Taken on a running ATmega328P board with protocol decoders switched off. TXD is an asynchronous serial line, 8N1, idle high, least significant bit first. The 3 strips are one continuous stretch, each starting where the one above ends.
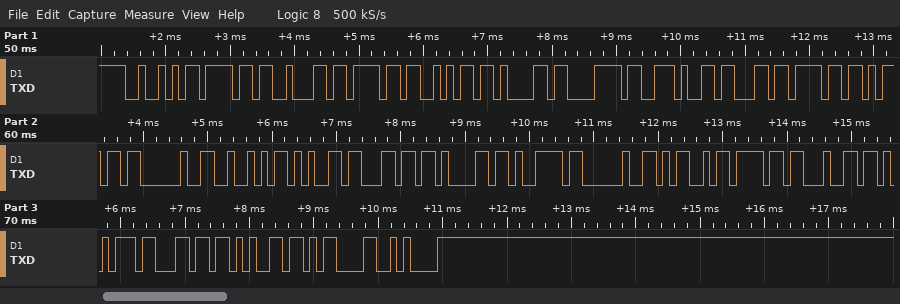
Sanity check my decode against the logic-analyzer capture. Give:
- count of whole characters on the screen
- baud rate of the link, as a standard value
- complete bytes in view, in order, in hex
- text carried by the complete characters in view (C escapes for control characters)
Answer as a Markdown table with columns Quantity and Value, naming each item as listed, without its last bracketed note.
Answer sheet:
| Quantity | Value |
|---|---|
| count of whole characters on the screen | 26 |
| baud rate of the link, as a standard value | 9600 baud |
| complete bytes in view, in order, in hex | 52 6F 62 6F 6A 61 78 2E 63 6F 6D 20 52 65 6C 61 79 20 4D 6F 64 75 6C 65 0D 0A |
| text carried by the complete characters in view | "Robojax.com Relay Module\r\n" |
